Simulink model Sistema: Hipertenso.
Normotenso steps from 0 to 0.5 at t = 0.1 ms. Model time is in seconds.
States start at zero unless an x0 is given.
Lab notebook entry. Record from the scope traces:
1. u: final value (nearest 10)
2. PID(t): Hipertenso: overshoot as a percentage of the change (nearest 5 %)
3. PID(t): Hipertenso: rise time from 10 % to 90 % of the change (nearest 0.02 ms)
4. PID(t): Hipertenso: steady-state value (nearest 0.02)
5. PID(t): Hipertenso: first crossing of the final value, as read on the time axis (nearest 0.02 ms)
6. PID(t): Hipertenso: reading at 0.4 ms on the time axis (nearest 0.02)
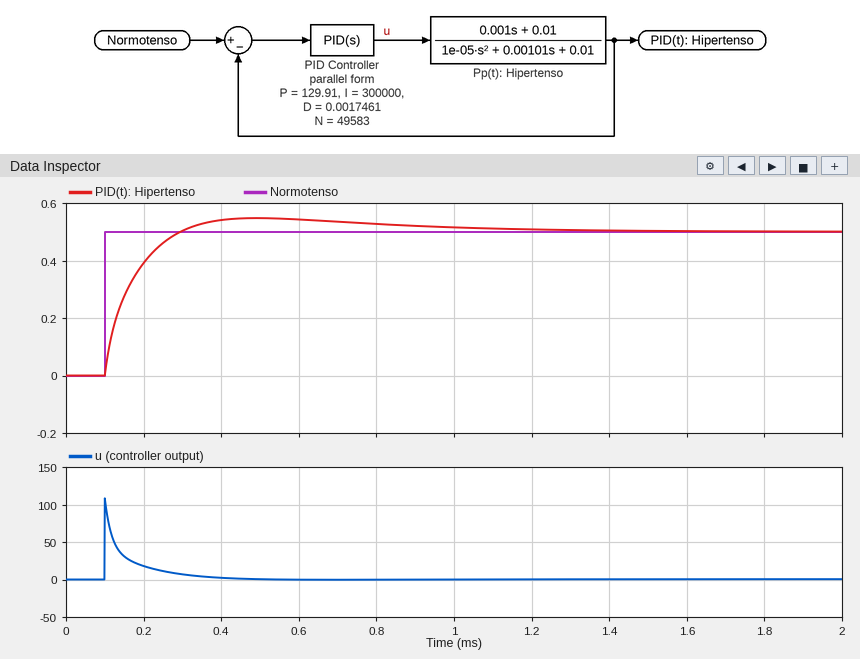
0
10 %
0.14 ms
0.50
0.30 ms
0.54
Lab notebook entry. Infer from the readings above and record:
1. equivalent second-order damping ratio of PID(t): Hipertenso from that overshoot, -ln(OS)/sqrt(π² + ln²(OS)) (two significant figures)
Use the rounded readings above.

0.59
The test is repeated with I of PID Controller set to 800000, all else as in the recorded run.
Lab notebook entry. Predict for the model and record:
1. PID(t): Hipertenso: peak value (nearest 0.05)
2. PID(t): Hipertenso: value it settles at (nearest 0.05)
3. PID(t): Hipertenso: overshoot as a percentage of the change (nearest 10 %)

0.60
0.50
20 %
